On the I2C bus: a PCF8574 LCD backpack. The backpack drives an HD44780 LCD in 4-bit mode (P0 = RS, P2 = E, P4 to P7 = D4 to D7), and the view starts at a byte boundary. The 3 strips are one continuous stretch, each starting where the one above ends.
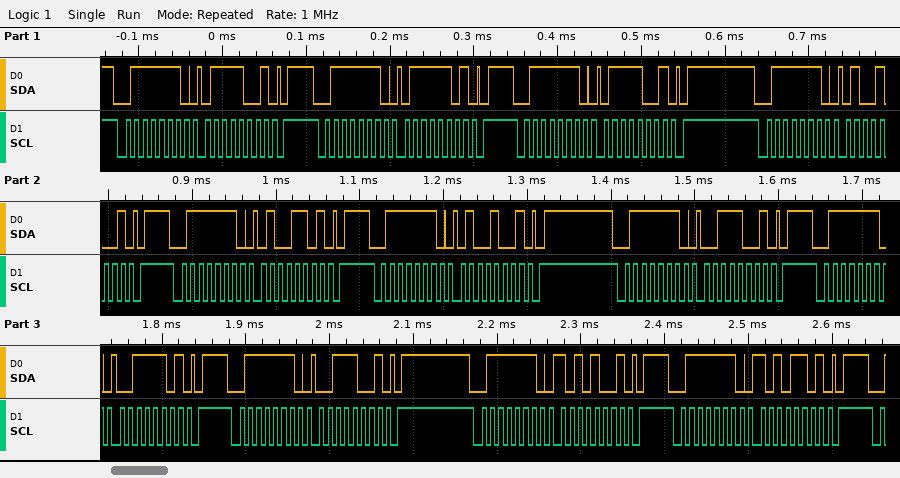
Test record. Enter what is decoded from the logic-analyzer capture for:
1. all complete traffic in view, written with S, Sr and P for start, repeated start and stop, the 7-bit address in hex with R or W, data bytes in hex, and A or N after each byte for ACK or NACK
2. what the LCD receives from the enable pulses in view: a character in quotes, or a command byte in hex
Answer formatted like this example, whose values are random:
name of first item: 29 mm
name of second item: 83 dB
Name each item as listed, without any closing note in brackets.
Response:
all complete traffic in view, written with S, Sr and P for start, repeated start and stop, the 7-bit address in hex with R or W, data bytes in hex, and A or N after each byte for ACK or NACK: S 3FW A 79 A P S 3FW A 7D A P S 3FW A 79 A P S 3FW A 49 A P S 3FW A 4D A P S 3FW A 49 A P S 3FW A 39 A P S 3FW A 3D A P S 3FW A 39 A P S 3FW A A9 A P S 3FW A AD A P
what the LCD receives from the enable pulses in view: a character in quotes, or a command byte in hex: 't'
